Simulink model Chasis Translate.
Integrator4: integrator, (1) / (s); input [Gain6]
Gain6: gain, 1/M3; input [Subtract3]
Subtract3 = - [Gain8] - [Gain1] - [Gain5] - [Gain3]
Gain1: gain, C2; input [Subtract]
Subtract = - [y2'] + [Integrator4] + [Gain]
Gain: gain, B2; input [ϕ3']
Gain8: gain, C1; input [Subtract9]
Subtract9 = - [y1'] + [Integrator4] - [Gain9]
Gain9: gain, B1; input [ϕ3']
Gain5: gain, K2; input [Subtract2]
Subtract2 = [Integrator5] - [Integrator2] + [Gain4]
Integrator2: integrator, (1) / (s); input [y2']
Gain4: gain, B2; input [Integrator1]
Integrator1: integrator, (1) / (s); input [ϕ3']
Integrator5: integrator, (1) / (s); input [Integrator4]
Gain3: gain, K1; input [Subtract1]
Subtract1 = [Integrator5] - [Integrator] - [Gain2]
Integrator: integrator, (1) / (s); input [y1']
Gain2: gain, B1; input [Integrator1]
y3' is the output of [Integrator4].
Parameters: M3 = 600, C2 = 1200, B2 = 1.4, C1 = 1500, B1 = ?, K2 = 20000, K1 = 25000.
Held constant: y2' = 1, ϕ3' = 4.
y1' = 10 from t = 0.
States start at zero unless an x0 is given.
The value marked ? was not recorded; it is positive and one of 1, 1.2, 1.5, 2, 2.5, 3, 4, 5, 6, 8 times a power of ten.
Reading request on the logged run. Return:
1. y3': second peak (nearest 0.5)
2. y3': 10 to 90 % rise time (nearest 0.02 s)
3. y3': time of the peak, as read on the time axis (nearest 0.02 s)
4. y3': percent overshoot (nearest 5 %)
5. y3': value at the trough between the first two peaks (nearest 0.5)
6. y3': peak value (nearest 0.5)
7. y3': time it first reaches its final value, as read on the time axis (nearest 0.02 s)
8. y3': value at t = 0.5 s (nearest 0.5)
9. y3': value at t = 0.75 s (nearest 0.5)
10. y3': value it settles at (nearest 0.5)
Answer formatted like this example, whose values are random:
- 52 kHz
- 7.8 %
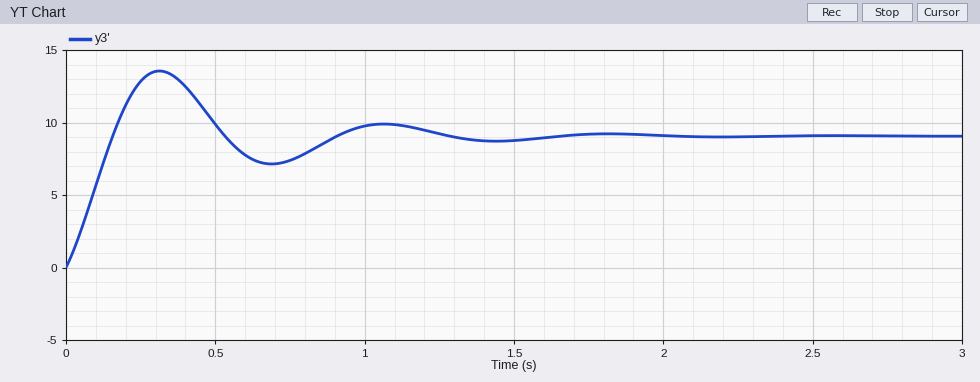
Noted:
- 10.0
- 0.12 s
- 0.32 s
- 50 %
- 7.0
- 13.5
- 0.16 s
- 10.0
- 7.5
- 9.0
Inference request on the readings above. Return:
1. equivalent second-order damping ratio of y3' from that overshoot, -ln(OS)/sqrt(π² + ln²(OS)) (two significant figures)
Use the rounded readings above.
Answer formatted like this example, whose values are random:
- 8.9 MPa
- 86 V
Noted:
- 0.22
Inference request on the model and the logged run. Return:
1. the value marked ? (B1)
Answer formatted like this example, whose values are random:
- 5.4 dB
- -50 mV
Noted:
- 2.5
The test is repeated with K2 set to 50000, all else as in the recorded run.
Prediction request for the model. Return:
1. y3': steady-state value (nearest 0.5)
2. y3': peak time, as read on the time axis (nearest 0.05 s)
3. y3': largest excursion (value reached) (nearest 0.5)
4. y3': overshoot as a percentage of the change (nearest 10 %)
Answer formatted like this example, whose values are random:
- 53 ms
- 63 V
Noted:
- 3.5
- 0.20 s
- 6.5
- 80 %
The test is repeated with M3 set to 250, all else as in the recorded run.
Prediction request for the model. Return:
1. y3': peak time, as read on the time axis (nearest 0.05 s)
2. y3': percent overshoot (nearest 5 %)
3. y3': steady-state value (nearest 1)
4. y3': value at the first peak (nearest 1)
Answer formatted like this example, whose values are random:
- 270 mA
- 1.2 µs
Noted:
- 0.20 s
- 35 %
- 9
- 12
